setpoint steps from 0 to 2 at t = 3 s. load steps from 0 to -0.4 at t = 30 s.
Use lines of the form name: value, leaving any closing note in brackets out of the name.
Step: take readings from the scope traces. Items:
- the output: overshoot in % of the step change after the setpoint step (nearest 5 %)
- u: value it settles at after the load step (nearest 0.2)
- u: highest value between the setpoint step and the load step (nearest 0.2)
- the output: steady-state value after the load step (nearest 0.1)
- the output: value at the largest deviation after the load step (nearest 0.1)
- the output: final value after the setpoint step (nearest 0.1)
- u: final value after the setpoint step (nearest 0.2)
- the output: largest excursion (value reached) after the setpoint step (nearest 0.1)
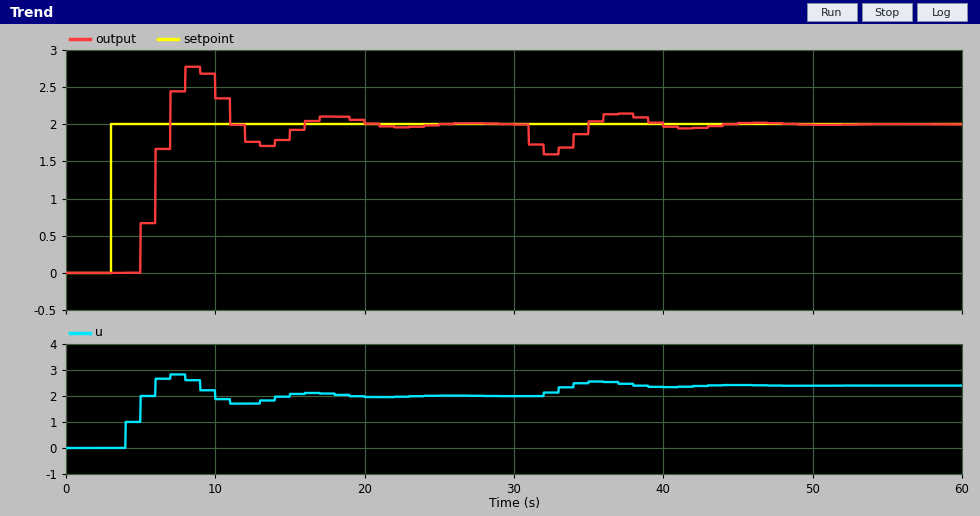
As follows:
the output: overshoot in % of the step change after the setpoint step: 40 %
u: value it settles at after the load step: 2.4
u: highest value between the setpoint step and the load step: 2.8
the output: steady-state value after the load step: 2.0
the output: value at the largest deviation after the load step: 1.6
the output: final value after the setpoint step: 2.0
u: final value after the setpoint step: 2.0
the output: largest excursion (value reached) after the setpoint step: 2.8
